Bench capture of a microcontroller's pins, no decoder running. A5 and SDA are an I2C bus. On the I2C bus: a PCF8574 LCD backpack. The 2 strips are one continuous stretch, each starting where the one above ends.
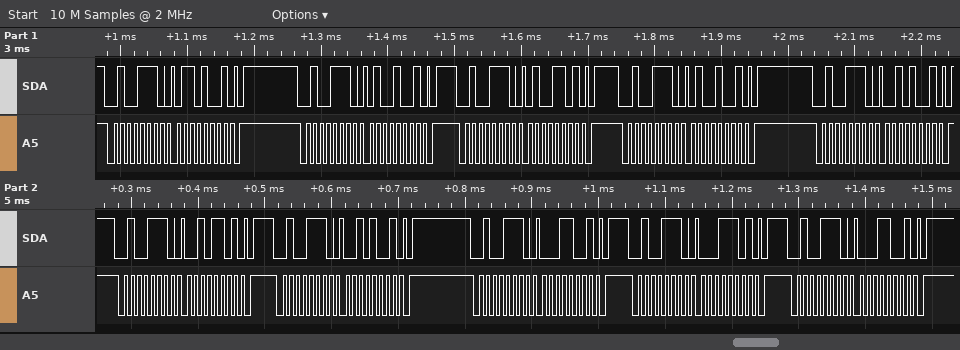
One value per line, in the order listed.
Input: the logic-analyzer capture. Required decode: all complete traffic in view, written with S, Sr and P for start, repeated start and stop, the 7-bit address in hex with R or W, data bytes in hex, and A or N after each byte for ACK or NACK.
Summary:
S 27W A 69 A P S 27W A 49 A P S 27W A 4D A P S 27W A 49 A P S 27W A 29 A P S 27W A 2D A P S 27W A 29 A P S 27W A 19 A P S 27W A 1D A P S 27W A 19 A P
